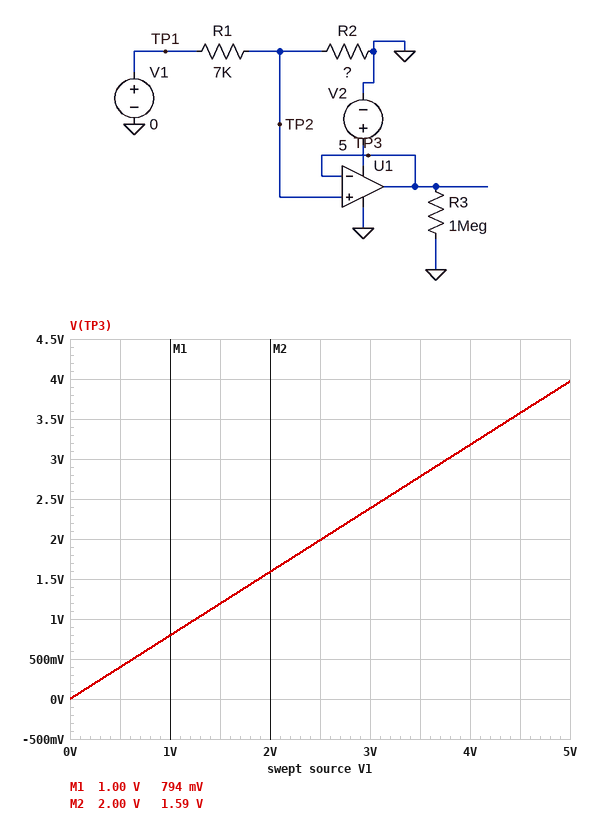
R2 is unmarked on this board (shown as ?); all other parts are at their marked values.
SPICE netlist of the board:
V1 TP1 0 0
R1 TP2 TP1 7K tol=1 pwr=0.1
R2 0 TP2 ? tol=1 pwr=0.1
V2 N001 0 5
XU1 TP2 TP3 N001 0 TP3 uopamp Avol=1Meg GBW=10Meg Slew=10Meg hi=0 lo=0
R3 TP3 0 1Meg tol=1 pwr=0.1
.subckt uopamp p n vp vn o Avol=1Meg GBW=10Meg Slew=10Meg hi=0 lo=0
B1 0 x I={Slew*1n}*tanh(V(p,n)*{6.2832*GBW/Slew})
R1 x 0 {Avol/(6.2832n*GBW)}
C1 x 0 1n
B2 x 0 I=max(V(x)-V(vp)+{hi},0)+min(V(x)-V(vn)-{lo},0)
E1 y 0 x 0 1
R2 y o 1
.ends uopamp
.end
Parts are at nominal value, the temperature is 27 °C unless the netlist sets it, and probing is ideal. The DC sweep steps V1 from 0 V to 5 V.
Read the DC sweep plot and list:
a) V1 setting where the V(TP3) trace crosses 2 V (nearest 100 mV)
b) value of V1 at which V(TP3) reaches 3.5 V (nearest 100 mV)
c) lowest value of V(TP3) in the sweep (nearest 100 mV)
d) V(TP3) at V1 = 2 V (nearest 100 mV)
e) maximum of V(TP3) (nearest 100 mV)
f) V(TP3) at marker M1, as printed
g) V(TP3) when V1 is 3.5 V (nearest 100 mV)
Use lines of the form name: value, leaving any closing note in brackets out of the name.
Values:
V1 setting where the V(TP3) trace crosses 2 V: 2.5 V
value of V1 at which V(TP3) reaches 3.5 V: 4.4 V
lowest value of V(TP3) in the sweep: 0 V
V(TP3) at V1 = 2 V: 1.6 V
maximum of V(TP3): 4.0 V
V(TP3) at marker M1, as printed: 794 mV
V(TP3) when V1 is 3.5 V: 2.8 V
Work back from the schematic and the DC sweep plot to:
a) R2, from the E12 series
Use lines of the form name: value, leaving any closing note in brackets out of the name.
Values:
R2, from the E12 series: 27 kΩ
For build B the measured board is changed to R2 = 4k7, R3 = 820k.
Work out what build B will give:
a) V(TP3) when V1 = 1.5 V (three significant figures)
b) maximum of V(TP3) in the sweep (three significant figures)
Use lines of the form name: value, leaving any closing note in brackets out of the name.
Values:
V(TP3) when V1 = 1.5 V: 603 mV
maximum of V(TP3) in the sweep: 2.01 V
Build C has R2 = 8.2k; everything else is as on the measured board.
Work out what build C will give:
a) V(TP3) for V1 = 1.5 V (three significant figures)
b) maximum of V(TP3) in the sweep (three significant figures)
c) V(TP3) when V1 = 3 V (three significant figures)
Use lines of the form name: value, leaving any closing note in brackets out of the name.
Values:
V(TP3) for V1 = 1.5 V: 809 mV
maximum of V(TP3) in the sweep: 2.70 V
V(TP3) when V1 = 3 V: 1.62 V
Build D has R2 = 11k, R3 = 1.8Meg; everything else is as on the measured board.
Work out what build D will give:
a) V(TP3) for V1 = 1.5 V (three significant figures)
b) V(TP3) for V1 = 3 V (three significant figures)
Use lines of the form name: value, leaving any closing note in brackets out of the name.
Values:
V(TP3) for V1 = 1.5 V: 917 mV
V(TP3) for V1 = 3 V: 1.83 V
